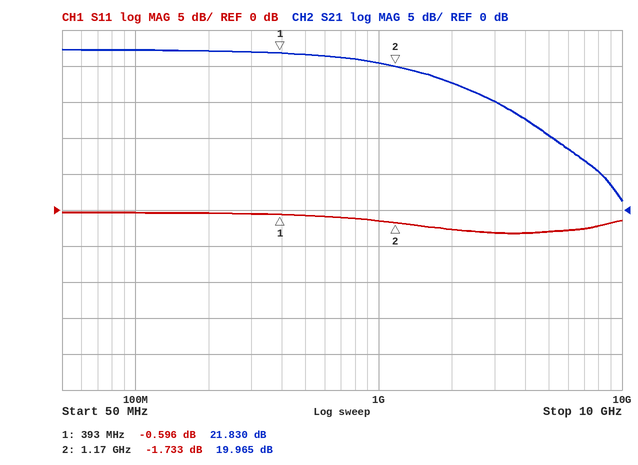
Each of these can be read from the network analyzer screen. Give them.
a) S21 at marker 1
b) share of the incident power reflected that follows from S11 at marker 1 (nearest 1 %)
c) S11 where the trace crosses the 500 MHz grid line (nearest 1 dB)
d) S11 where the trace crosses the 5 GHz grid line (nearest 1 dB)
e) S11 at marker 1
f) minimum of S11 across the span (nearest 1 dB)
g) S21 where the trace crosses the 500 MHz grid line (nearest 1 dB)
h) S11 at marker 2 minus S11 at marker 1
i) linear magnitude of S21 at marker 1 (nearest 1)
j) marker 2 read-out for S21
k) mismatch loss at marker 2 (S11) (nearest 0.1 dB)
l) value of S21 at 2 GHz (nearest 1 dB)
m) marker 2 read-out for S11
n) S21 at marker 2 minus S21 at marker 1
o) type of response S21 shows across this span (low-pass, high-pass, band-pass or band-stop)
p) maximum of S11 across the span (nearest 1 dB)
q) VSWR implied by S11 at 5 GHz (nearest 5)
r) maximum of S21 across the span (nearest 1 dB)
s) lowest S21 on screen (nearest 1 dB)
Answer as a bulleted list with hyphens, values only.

- 21.830 dB
- 87 %
- -1 dB
- -3 dB
- -0.596 dB
- -3 dB
- 22 dB
- -1.137 dB
- 12
- 19.965 dB
- 4.8 dB
- 18 dB
- -1.733 dB
- -1.865 dB
- low-pass
- 0 dB
- 5
- 22 dB
- 1 dB
